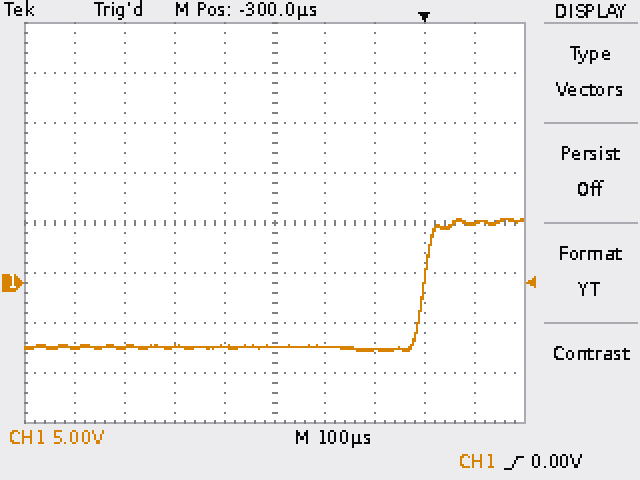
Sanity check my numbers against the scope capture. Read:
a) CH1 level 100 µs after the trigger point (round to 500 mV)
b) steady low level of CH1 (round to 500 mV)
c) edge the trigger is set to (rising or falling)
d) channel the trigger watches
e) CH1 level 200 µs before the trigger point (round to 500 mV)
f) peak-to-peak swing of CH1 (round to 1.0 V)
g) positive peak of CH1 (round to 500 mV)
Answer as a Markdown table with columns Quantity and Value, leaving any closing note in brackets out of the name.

| Quantity | Value |
|---|---|
| CH1 level 100 µs after the trigger point | 6.0 V |
| steady low level of CH1 | -6.5 V |
| edge the trigger is set to | rising |
| channel the trigger watches | CH1 |
| CH1 level 200 µs before the trigger point | -6.5 V |
| peak-to-peak swing of CH1 | 13.0 V |
| positive peak of CH1 | 6.5 V |
